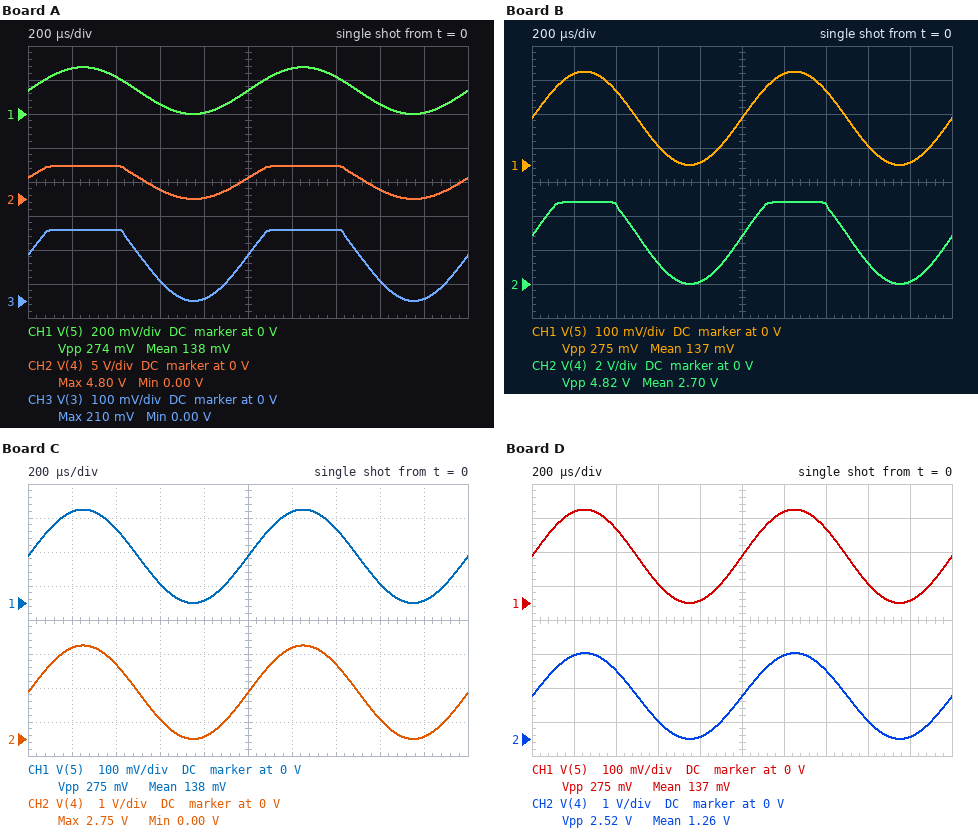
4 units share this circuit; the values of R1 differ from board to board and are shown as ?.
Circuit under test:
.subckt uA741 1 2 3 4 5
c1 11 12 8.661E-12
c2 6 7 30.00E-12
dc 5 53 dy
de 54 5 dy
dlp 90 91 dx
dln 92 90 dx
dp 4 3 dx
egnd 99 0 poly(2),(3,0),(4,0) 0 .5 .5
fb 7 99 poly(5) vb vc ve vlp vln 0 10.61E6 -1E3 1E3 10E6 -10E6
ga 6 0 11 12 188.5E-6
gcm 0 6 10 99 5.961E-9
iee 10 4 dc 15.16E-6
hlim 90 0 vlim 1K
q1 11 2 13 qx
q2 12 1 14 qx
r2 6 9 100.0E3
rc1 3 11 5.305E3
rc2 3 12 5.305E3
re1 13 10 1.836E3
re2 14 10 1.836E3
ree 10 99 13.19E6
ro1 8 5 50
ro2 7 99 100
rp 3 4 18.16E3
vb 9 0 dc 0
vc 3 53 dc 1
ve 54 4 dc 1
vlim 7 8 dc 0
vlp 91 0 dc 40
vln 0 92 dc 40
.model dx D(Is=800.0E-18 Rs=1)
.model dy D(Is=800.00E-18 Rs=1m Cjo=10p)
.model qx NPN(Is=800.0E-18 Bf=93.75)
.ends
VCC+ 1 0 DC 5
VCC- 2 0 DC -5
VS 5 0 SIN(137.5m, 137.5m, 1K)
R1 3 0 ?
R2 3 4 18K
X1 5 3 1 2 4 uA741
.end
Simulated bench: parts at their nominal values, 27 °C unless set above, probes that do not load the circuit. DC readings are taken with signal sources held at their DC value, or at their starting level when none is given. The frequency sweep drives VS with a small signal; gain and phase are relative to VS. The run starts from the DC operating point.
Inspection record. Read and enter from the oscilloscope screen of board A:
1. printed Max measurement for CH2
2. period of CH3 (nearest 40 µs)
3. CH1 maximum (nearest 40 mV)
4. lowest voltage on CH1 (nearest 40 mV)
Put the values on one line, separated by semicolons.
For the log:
4.80 V; 1.00 ms; 280 mV; 0 V
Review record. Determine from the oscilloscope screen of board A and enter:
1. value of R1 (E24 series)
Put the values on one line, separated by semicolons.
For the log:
820 Ω
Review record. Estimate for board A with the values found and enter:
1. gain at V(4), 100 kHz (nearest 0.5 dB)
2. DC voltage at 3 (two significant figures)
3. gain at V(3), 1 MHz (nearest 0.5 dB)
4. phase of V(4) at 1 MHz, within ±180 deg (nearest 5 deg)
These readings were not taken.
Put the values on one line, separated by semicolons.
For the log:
19.5 dB; 140 mV; -28.5 dB; -120 deg
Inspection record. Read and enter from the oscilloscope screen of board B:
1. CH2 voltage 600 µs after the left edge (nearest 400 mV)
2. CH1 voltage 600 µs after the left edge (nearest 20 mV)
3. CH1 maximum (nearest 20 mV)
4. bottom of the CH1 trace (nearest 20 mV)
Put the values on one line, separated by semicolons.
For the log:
1.2 V; 60 mV; 280 mV; 0 V
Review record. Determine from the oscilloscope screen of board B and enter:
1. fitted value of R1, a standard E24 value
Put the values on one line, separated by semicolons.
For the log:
910 Ω
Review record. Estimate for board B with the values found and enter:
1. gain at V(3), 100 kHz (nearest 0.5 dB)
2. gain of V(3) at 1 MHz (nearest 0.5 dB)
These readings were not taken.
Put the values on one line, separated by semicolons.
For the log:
-7.0 dB; -27.5 dB
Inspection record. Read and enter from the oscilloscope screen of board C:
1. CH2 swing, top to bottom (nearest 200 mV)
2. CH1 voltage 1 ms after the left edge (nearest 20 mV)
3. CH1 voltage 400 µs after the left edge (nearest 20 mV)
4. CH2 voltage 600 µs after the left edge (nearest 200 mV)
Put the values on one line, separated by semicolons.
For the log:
2.8 V; 140 mV; 220 mV; 600 mV
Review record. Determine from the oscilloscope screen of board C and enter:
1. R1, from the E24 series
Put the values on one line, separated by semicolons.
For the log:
2 kΩ
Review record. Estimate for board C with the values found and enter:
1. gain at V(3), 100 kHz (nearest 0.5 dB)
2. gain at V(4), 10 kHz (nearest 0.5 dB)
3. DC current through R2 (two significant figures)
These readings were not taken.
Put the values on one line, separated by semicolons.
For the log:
-3.0 dB; 20.0 dB; 69 µA
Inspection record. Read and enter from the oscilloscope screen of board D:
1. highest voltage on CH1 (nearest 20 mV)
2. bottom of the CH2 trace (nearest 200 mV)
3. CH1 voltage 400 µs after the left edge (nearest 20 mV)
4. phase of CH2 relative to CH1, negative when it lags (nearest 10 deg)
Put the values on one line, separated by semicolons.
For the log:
280 mV; 0 V; 220 mV; 0 deg
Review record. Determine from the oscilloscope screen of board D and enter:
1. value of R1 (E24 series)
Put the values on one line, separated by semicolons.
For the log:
2.2 kΩ
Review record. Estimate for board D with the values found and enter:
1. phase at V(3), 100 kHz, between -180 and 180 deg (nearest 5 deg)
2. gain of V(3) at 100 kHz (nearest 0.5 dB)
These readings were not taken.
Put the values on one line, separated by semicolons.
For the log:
-45 deg; -2.5 dB
